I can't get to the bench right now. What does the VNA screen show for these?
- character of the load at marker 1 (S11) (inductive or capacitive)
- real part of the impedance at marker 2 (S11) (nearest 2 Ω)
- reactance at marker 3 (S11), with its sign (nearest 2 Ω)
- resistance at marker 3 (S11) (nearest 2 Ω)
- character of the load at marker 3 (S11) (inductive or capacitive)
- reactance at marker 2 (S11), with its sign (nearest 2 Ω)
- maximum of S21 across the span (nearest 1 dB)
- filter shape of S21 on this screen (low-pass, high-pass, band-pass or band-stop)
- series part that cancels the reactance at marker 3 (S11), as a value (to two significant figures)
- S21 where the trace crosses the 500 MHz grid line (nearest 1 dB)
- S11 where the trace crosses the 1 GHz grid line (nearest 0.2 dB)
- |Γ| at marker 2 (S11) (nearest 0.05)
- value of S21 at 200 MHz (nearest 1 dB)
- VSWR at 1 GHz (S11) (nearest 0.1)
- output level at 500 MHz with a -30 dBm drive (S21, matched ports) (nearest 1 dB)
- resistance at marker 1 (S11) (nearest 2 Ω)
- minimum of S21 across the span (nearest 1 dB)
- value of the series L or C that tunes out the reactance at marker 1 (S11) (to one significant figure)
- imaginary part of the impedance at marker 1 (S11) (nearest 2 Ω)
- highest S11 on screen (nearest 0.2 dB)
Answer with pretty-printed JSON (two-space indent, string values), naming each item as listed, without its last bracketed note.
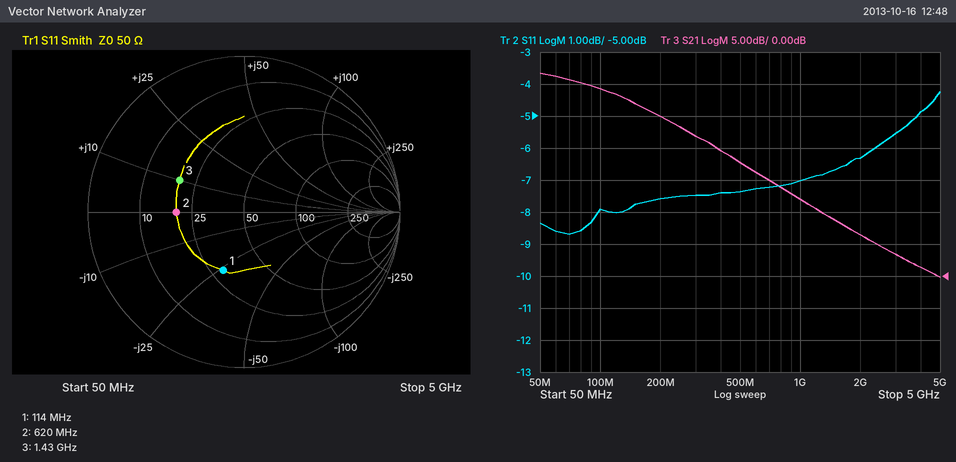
{
  "character of the load at marker 1 (S11)": "capacitive",
  "real part of the impedance at marker 2 (S11)": "20 Ω",
  "reactance at marker 3 (S11), with its sign": "+10 Ω",
  "resistance at marker 3 (S11)": "20 Ω",
  "character of the load at marker 3 (S11)": "inductive",
  "reactance at marker 2 (S11), with its sign": "0 Ω",
  "maximum of S21 across the span": "32 dB",
  "filter shape of S21 on this screen": "low-pass",
  "series part that cancels the reactance at marker 3 (S11), as a value": "11 pF",
  "S21 where the trace crosses the 500 MHz grid line": "18 dB",
  "S11 where the trace crosses the 1 GHz grid line": "-7.0 dB",
  "|Γ| at marker 2 (S11)": "0.45",
  "value of S21 at 200 MHz": "25 dB",
  "VSWR at 1 GHz (S11)": "2.6",
  "output level at 500 MHz with a -30 dBm drive (S21, matched ports)": "-12 dBm",
  "resistance at marker 1 (S11)": "30 Ω",
  "minimum of S21 across the span": "0 dB",
  "value of the series L or C that tunes out the reactance at marker 1 (S11)": "40 nH",
  "imaginary part of the impedance at marker 1 (S11)": "-26 Ω",
  "highest S11 on screen": "-4.2 dB"
}
